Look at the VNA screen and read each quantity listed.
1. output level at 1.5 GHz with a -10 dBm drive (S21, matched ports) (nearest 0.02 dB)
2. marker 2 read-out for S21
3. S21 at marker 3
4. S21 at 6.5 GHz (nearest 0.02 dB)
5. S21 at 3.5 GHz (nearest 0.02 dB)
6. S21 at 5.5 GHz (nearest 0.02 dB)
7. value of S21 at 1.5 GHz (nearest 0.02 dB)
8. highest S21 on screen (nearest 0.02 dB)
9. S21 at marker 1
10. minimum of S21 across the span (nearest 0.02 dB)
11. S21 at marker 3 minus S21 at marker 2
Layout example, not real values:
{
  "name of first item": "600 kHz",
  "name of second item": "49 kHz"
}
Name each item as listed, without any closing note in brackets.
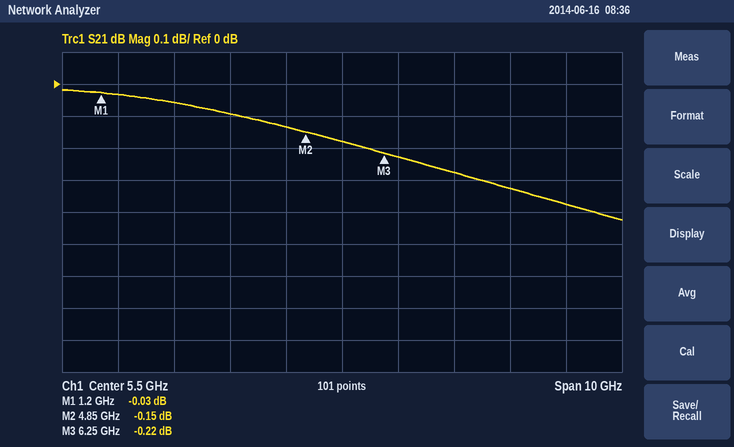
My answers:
{
  "output level at 1.5 GHz with a -10 dBm drive (S21, matched ports)": "-10.04 dBm",
  "marker 2 read-out for S21": "-0.15 dB",
  "S21 at marker 3": "-0.22 dB",
  "S21 at 6.5 GHz": "-0.22 dB",
  "S21 at 3.5 GHz": "-0.10 dB",
  "S21 at 5.5 GHz": "-0.18 dB",
  "value of S21 at 1.5 GHz": "-0.04 dB",
  "highest S21 on screen": "-0.02 dB",
  "S21 at marker 1": "-0.03 dB",
  "minimum of S21 across the span": "-0.42 dB",
  "S21 at marker 3 minus S21 at marker 2": "-0.07 dB"
}
